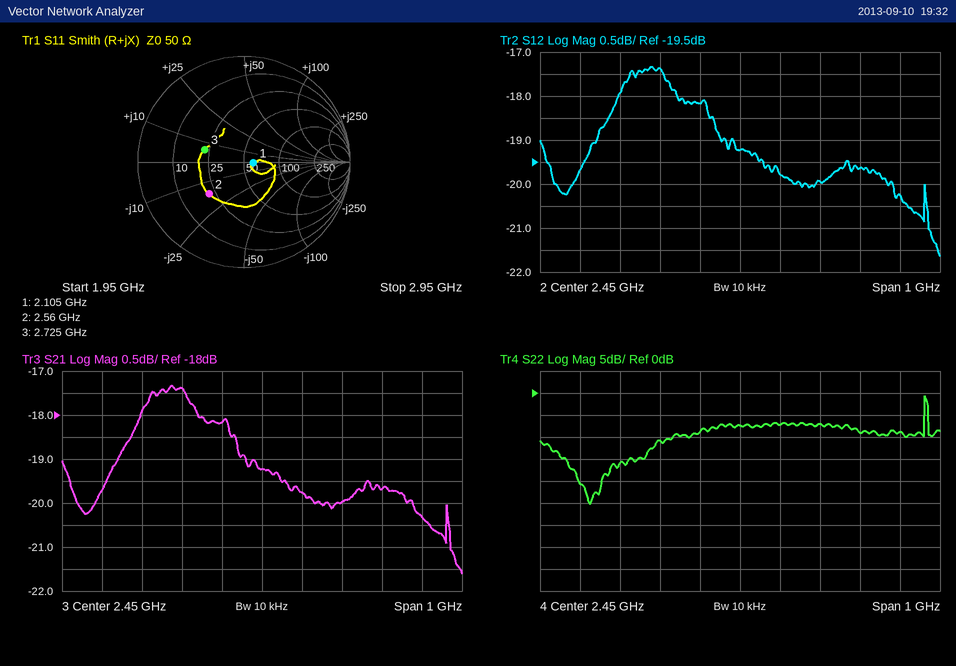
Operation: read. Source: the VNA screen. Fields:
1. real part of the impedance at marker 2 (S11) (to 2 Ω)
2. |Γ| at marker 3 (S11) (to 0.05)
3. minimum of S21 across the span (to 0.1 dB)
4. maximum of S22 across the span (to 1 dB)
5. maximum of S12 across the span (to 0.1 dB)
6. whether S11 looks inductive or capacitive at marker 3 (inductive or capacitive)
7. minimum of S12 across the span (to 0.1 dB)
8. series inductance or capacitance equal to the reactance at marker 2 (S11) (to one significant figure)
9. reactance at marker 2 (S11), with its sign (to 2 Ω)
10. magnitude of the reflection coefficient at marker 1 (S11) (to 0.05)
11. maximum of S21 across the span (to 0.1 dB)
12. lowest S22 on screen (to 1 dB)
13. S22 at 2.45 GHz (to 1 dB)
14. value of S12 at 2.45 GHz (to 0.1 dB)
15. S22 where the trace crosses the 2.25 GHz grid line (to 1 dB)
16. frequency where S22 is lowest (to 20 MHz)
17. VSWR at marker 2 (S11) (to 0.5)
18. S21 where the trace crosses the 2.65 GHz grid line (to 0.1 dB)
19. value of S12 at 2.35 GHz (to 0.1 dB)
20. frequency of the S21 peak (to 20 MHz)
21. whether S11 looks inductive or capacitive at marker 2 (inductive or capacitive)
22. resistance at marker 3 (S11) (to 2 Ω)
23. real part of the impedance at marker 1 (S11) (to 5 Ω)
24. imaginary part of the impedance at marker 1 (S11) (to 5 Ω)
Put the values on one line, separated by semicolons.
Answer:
22 Ω; 0.40; -21.6 dB; -1 dB; -17.3 dB; inductive; -21.6 dB; 4 pF; -16 Ω; 0.10; -17.3 dB; -25 dB; -7 dB; -19.2 dB; -11 dB; 2.08 GHz; 2.5; -20.0 dB; -18.2 dB; 2.22 GHz; capacitive; 22 Ω; 60 Ω; 0 Ω
